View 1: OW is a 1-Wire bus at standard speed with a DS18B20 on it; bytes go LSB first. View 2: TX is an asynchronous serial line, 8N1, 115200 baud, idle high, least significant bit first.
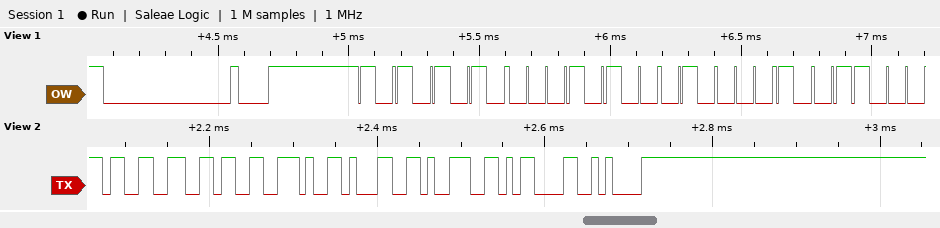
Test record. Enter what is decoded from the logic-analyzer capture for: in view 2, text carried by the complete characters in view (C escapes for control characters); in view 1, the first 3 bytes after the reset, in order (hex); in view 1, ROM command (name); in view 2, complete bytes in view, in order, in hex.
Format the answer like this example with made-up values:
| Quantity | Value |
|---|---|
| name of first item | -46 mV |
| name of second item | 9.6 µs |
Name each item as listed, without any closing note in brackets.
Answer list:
| Quantity | Value |
|---|---|
| in view 2, text carried by the complete characters in view | "36.19\r\n" |
| in view 1, the first 3 bytes after the reset, in order | 55 28 42 |
| in view 1, ROM command | Match ROM |
| in view 2, complete bytes in view, in order, in hex | 33 36 2E 31 39 0D 0A |
